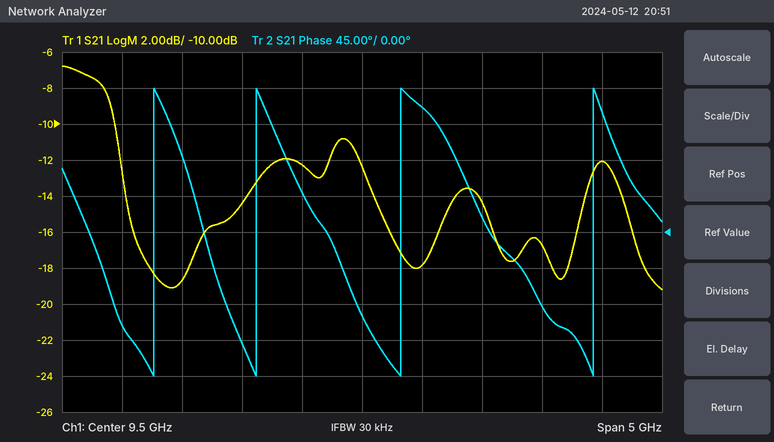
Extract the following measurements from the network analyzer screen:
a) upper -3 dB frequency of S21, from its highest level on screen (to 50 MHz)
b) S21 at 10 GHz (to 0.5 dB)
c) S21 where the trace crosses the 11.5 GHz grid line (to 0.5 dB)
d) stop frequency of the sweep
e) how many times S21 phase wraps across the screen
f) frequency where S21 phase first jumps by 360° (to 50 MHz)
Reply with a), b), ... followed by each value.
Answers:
a) 7.45 GHz
b) -18.0 dB
c) -12.0 dB
d) 12 GHz
e) 4
f) 7.75 GHz
